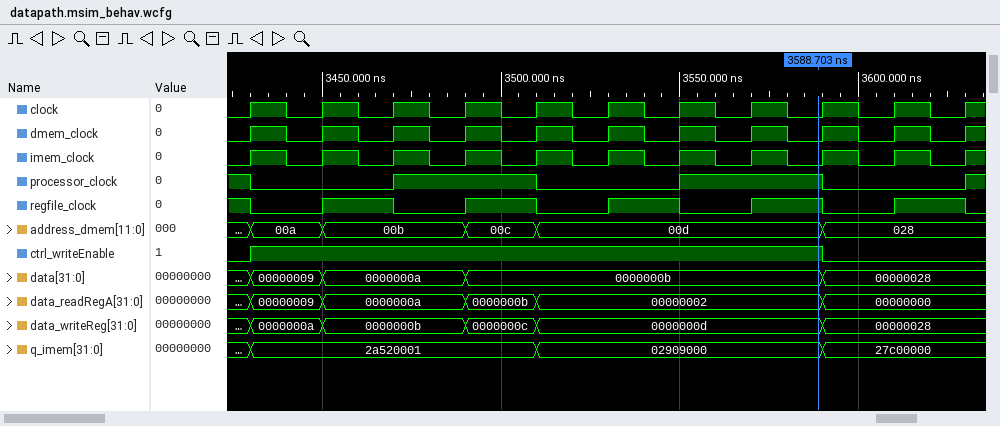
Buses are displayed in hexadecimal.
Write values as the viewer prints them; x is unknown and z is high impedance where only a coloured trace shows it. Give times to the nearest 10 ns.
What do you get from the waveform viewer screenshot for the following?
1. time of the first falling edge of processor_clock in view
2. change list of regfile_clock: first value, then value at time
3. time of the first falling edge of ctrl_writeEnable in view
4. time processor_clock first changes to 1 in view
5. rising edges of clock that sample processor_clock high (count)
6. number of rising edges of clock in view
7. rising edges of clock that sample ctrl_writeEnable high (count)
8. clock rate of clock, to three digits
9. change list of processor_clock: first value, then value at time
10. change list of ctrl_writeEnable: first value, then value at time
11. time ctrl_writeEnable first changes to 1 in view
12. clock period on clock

3430 ns
1, 0 at 3430 ns, 1 at 3450 ns, 0 at 3470 ns, 1 at 3490 ns, 0 at 3510 ns, 1 at 3530 ns, 0 at 3550 ns, 1 at 3570 ns, 0 at 3590 ns, 1 at 3610 ns, 0 at 3630 ns
3590 ns
3470 ns
5
11
8
50.0 MHz
1, 0 at 3430 ns, 1 at 3470 ns, 0 at 3510 ns, 1 at 3550 ns, 0 at 3590 ns, 1 at 3630 ns
0, 1 at 3430 ns, 0 at 3590 ns
3430 ns
20 ns
